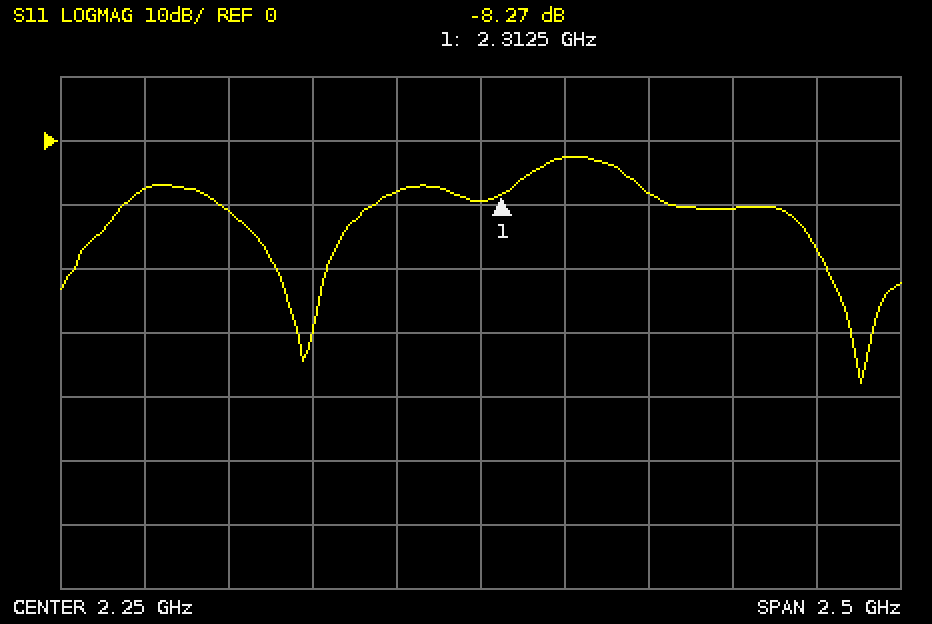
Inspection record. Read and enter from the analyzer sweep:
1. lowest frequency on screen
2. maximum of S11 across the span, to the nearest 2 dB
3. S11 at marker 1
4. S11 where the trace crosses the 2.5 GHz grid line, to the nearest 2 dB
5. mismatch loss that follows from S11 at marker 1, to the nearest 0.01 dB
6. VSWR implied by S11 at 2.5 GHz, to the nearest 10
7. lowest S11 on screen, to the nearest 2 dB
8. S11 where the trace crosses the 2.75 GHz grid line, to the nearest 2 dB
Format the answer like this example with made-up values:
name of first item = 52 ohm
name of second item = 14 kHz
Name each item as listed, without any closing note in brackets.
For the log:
lowest frequency on screen = 1 GHz
maximum of S11 across the span, to the nearest 2 dB = -2 dB
S11 at marker 1 = -8.27 dB
S11 where the trace crosses the 2.5 GHz grid line, to the nearest 2 dB = -2 dB
mismatch loss that follows from S11 at marker 1, to the nearest 0.01 dB = 0.70 dB
VSWR implied by S11 at 2.5 GHz, to the nearest 10 = 10
lowest S11 on screen, to the nearest 2 dB = -38 dB
S11 where the trace crosses the 2.75 GHz grid line, to the nearest 2 dB = -8 dB
